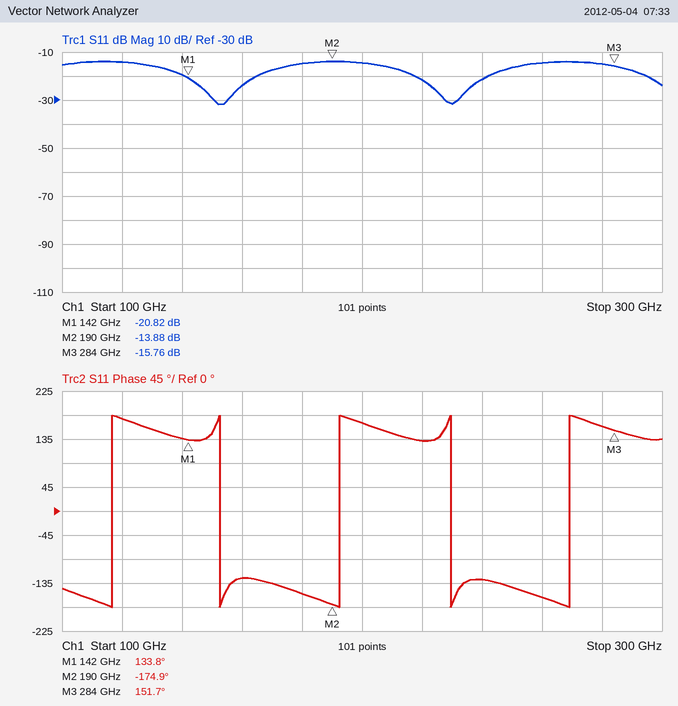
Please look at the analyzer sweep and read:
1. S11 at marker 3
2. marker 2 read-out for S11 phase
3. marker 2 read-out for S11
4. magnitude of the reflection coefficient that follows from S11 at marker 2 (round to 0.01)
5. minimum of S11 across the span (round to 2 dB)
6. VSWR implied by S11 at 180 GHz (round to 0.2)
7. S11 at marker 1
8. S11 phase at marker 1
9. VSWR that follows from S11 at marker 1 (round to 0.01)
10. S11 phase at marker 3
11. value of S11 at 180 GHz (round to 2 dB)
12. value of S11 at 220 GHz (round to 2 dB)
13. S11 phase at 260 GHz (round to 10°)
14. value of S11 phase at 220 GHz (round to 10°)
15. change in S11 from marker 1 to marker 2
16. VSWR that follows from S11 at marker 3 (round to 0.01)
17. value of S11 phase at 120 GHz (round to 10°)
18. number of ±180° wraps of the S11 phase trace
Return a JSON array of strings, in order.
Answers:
["-15.76 dB", "-174.9°", "-13.88 dB", "0.20", "-32 dB", "1.4", "-20.82 dB", "133.8°", "1.20", "151.7°", "-14 dB", "-22 dB", "-160°", "130°", "6.94 dB", "1.39", "170°", "5"]
